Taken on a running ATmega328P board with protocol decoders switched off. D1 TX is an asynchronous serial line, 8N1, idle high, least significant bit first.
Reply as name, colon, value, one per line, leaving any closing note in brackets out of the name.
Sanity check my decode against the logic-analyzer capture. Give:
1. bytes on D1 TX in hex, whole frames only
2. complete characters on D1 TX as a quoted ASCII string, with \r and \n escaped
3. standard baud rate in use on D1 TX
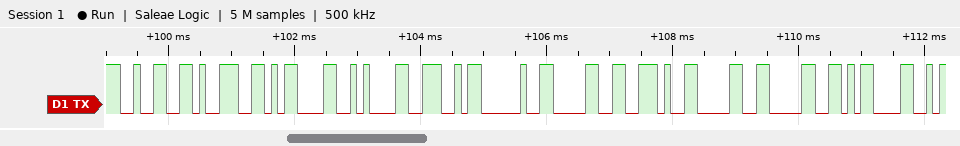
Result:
bytes on D1 TX in hex, whole frames only: 32 39 0D 0A 4E 20 30 2E 30 30 0D
complete characters on D1 TX as a quoted ASCII string, with \r and \n escaped: "29\r\nN 0.00\r"
standard baud rate in use on D1 TX: 9600 baud
